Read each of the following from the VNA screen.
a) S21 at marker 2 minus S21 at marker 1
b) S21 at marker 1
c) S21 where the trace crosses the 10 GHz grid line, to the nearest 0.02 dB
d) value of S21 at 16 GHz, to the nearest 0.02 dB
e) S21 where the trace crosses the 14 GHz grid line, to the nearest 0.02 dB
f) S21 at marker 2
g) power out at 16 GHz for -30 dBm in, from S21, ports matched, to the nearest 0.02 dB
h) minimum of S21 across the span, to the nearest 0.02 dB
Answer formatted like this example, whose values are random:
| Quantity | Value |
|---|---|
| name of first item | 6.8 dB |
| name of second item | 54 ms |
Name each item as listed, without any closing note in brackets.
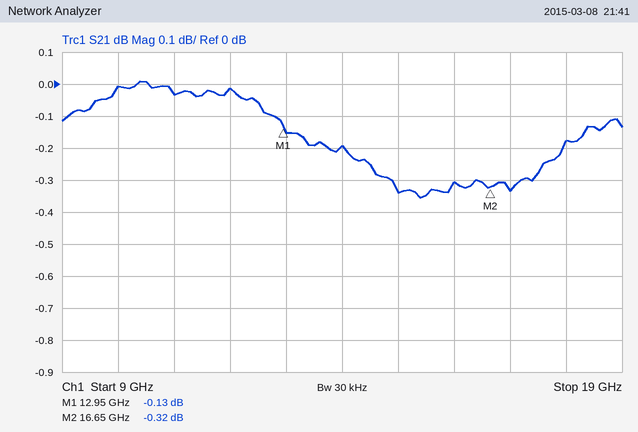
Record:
| Quantity | Value |
|---|---|
| S21 at marker 2 minus S21 at marker 1 | -0.19 dB |
| S21 at marker 1 | -0.13 dB |
| S21 where the trace crosses the 10 GHz grid line, to the nearest 0.02 dB | 0.00 dB |
| value of S21 at 16 GHz, to the nearest 0.02 dB | -0.30 dB |
| S21 where the trace crosses the 14 GHz grid line, to the nearest 0.02 dB | -0.20 dB |
| S21 at marker 2 | -0.32 dB |
| power out at 16 GHz for -30 dBm in, from S21, ports matched, to the nearest 0.02 dB | -30.30 dBm |
| minimum of S21 across the span, to the nearest 0.02 dB | -0.36 dB |
